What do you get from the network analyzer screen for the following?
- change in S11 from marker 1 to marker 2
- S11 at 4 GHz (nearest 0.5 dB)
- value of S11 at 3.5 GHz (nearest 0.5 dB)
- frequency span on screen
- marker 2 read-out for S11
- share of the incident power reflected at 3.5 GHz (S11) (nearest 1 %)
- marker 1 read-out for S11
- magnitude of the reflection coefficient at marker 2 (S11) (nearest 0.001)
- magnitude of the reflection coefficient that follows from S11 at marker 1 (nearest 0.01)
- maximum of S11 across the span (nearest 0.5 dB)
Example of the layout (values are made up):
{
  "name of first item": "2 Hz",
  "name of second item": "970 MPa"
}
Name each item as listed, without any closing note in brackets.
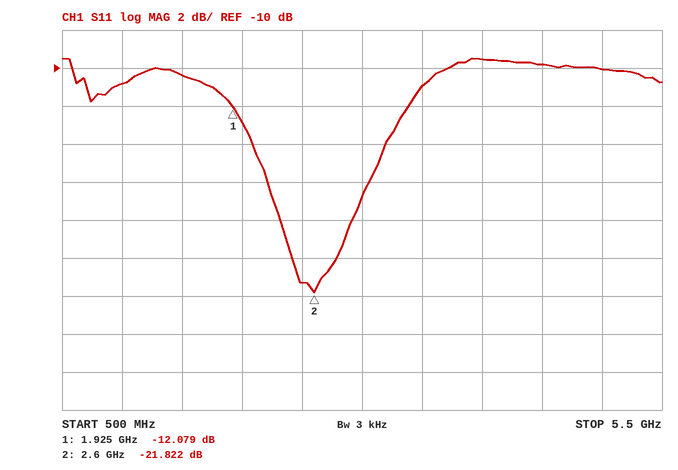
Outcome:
{
  "change in S11 from marker 1 to marker 2": "-9.743 dB",
  "S11 at 4 GHz": "-9.5 dB",
  "value of S11 at 3.5 GHz": "-11.0 dB",
  "frequency span on screen": "5 GHz",
  "marker 2 read-out for S11": "-21.822 dB",
  "share of the incident power reflected at 3.5 GHz (S11)": "8 %",
  "marker 1 read-out for S11": "-12.079 dB",
  "magnitude of the reflection coefficient at marker 2 (S11)": "0.081",
  "magnitude of the reflection coefficient that follows from S11 at marker 1": "0.25",
  "maximum of S11 across the span": "-9.5 dB"
}
